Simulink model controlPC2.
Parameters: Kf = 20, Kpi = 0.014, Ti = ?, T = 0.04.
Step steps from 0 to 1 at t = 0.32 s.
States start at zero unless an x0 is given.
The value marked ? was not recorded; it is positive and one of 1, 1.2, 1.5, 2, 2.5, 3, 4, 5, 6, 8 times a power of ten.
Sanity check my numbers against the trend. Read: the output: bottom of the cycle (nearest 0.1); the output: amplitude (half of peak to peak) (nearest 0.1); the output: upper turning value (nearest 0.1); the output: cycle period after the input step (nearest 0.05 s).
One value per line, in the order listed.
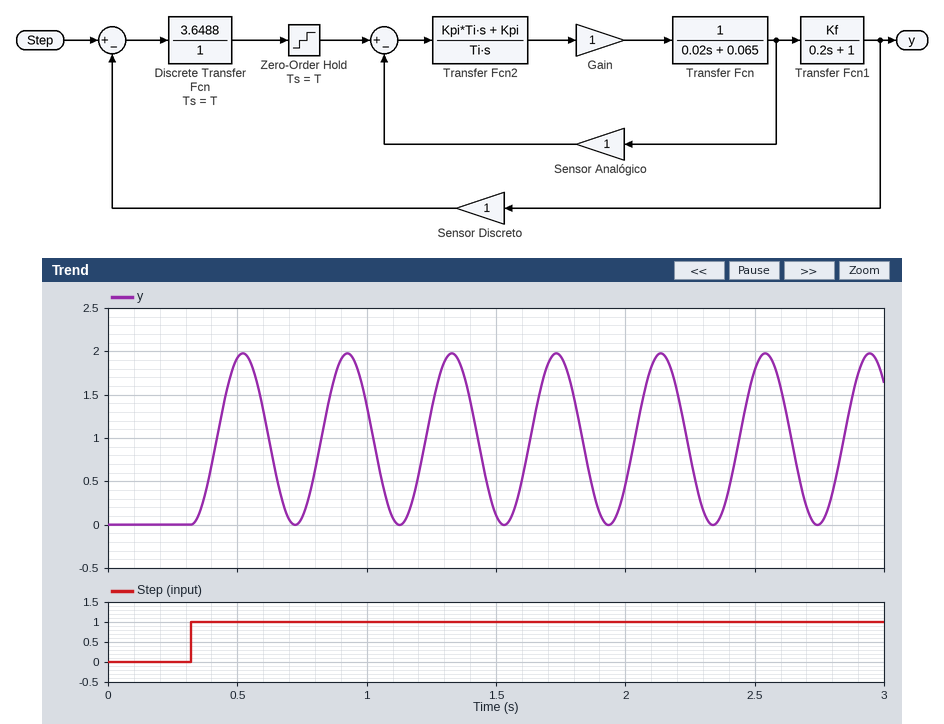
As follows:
0.0
1.0
2.0
0.40 s
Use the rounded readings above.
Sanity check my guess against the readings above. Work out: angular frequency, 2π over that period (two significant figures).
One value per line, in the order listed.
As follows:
16 rad/s
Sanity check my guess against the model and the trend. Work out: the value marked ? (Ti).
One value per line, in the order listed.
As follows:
0.25
